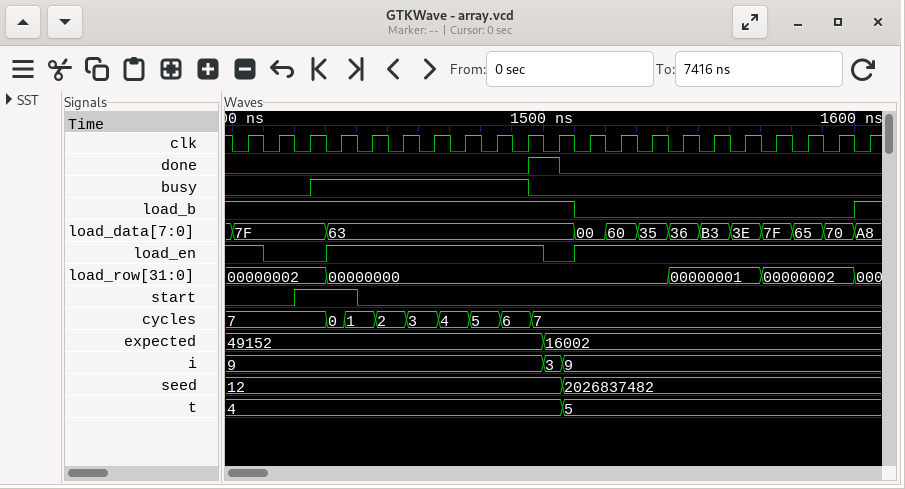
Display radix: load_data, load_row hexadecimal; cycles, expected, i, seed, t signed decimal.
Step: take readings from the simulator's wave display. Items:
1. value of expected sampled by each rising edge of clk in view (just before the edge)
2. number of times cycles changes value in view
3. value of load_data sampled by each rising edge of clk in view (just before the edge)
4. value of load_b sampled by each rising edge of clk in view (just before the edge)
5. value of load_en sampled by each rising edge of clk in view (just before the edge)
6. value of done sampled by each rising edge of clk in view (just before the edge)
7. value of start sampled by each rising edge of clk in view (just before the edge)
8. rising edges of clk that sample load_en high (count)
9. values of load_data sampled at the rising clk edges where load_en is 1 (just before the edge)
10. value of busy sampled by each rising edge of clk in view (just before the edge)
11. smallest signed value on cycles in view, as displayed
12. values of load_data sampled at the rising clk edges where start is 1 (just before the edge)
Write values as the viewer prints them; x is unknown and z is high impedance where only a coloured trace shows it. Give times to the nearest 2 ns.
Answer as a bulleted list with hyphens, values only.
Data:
- 49152, 49152, 49152, 49152, 49152, 49152, 49152, 49152, 49152, 49152, 16002, 16002, 16002, 16002, 16002, 16002, 16002, 16002, 16002, 16002, 16002
- 8
- 7F, 7F, 7F, 63, 63, 63, 63, 63, 63, 63, 63, 00, 60, 35, 36, B3, 3E, 7F, 65, 70, A8
- 1 1 1 1 1 1 1 1 1 1 1 0 0 0 0 0 0 0 0 0 1
- 1 0 0 1 1 1 1 1 1 1 0 1 1 1 1 1 1 1 1 1 1
- 0 0 0 0 0 0 0 0 0 0 1 0 0 0 0 0 0 0 0 0 0
- 0 0 1 1 0 0 0 0 0 0 0 0 0 0 0 0 0 0 0 0 0
- 18
- 7F, 63, 63, 63, 63, 63, 63, 63, 00, 60, 35, 36, B3, 3E, 7F, 65, 70, A8
- 0 0 0 1 1 1 1 1 1 1 0 0 0 0 0 0 0 0 0 0 0
- 0
- 7F, 63
